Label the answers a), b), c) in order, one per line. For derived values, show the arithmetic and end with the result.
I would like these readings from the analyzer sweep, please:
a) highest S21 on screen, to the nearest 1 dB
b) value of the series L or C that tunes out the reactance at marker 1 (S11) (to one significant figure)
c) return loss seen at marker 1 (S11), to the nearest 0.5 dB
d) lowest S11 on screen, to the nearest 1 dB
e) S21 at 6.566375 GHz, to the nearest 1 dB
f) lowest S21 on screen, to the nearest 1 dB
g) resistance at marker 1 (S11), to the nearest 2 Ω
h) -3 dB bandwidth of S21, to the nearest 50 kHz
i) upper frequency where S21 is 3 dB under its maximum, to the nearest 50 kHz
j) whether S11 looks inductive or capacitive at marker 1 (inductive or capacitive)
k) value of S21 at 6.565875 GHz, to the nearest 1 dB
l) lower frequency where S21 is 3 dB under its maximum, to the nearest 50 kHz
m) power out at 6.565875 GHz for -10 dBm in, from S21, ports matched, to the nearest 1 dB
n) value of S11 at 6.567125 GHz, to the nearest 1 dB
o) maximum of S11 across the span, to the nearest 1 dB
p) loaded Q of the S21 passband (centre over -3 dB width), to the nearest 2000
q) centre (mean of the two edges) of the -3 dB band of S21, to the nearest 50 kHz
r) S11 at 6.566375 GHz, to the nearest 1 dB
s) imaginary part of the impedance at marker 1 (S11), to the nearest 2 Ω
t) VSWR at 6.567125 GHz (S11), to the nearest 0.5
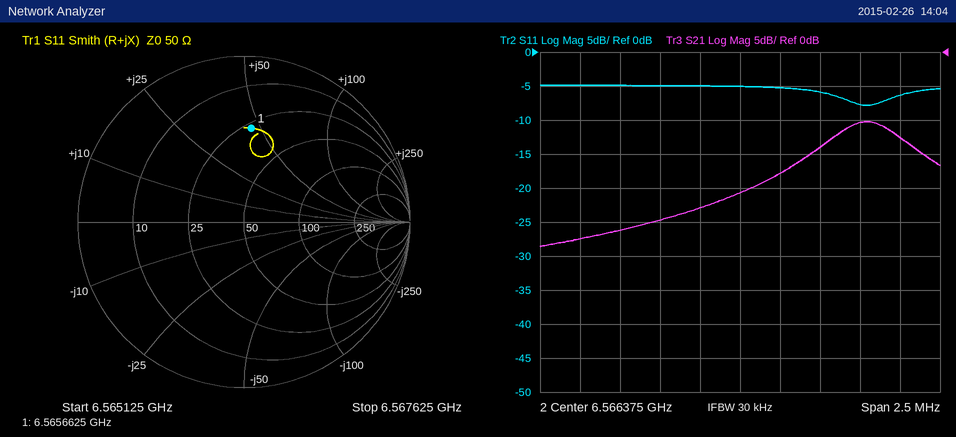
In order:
a) -10 dB
b) C = 1/(2π × 6.5656625 GHz × 46 Ω) ≈ 527 fF, so 500 fF to one significant figure
c) 5.0 dB
d) -8 dB
e) -21 dB
f) -29 dB
g) 28 Ω
h) 6.56740 GHz − 6.56690 GHz = 500 kHz
i) 6.56740 GHz
j) inductive
k) -25 dB
l) 6.56690 GHz
m) -10 dBm + (-25 dB) = -35 dBm
n) -8 dB
o) -5 dB
p) 6.56715 GHz / 500 kHz ≈ 13134, so 14000 to the nearest 2000
q) 6.56715 GHz
r) -5 dB
s) +46 Ω
t) |Γ| = 10^(-8/20) = 0.3981; VSWR = (1 + 0.3981)/(1 − 0.3981) ≈ 2.32, so 2.5 to the nearest 0.5
